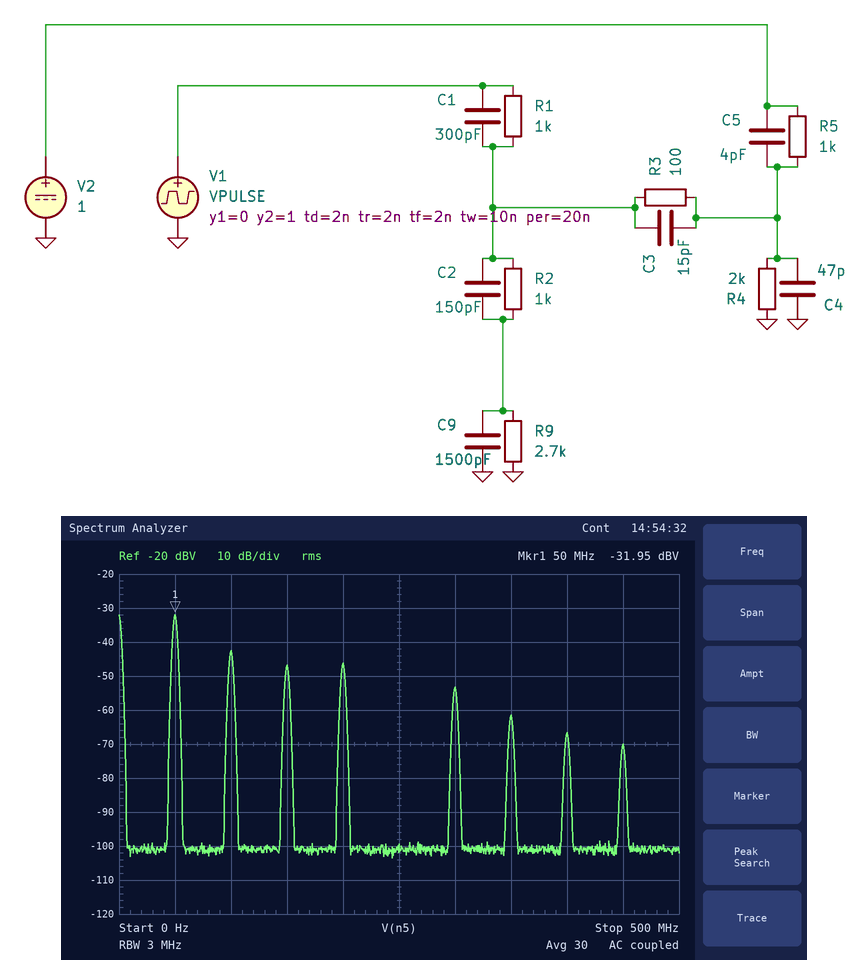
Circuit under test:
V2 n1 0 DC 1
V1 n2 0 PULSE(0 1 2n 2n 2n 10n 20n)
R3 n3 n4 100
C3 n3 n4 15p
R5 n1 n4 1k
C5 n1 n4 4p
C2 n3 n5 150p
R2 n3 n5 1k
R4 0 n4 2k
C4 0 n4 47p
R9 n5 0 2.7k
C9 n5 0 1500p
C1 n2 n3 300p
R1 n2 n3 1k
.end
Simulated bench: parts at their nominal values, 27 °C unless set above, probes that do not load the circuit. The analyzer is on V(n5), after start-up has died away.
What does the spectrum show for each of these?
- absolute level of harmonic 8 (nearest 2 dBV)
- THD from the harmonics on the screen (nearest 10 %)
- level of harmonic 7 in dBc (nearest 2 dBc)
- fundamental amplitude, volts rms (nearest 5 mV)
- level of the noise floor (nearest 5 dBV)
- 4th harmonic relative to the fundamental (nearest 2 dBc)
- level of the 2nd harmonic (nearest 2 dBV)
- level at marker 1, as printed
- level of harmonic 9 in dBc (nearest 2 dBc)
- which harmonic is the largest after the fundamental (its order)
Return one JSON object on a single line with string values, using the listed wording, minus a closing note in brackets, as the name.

{"absolute level of harmonic 8": "-66 dBV", "THD from the harmonics on the screen": "40 %", "level of harmonic 7 in dBc": "-30 dBc", "fundamental amplitude, volts rms": "25 mV", "level of the noise floor": "-100 dBV", "4th harmonic relative to the fundamental": "-14 dBc", "level of the 2nd harmonic": "-42 dBV", "level at marker 1, as printed": "-31.95 dBV", "level of harmonic 9 in dBc": "-38 dBc", "which harmonic is the largest after the fundamental": "2"}
